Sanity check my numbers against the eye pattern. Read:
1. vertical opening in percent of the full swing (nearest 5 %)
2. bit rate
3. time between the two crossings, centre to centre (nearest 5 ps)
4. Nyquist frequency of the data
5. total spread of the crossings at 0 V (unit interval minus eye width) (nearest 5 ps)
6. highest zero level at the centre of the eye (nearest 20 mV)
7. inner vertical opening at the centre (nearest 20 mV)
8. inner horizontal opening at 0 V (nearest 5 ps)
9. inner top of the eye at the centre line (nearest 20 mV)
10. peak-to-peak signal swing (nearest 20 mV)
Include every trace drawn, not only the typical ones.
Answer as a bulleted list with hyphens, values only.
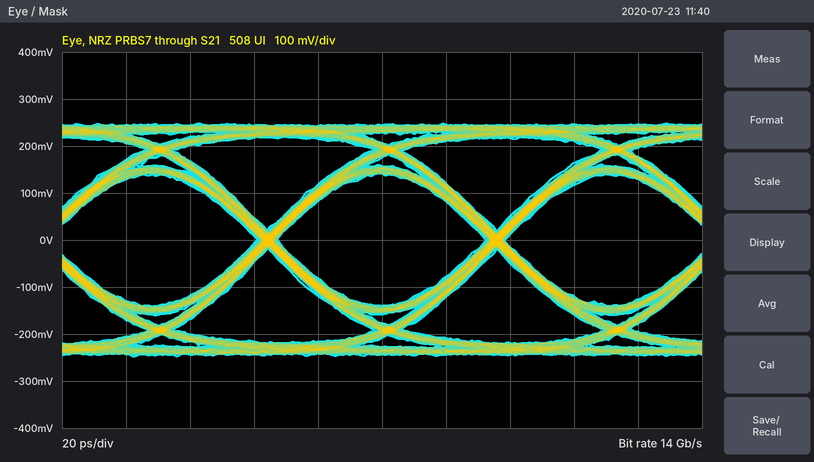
- 55 %
- 14 Gb/s
- 70 ps
- 7 GHz
- 5 ps
- -140 mV
- 280 mV
- 65 ps
- 140 mV
- 500 mV
